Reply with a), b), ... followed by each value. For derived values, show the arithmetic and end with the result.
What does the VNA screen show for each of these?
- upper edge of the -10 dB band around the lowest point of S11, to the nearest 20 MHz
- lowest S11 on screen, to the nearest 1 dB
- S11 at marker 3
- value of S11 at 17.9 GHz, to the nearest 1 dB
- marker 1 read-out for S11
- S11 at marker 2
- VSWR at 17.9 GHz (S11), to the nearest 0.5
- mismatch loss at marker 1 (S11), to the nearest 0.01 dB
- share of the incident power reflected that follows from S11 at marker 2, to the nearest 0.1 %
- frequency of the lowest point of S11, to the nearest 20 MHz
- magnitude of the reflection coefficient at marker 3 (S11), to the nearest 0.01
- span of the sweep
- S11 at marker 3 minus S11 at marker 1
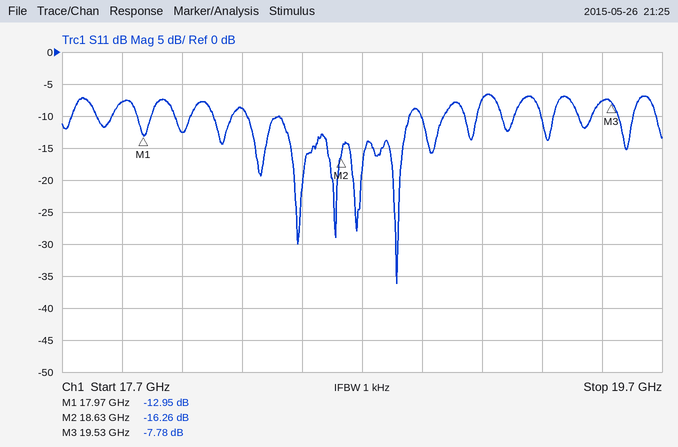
a) 18.86 GHz
b) -36 dB
c) -7.78 dB
d) -8 dB
e) -12.95 dB
f) -16.26 dB
g) |Γ| = 10^(-8/20) = 0.3981; VSWR = (1 + 0.3981)/(1 − 0.3981) ≈ 2.32, so 2.5 to the nearest 0.5
h) −10 log10(1 − 10^(-12.95/10)) ≈ 0.23 dB
i) 10^(-16.26/10) ≈ 2.4 %
j) 18.82 GHz
k) 10^(-7.78/20) ≈ 0.41
l) 2 GHz
m) -7.78 − (-12.95) = 5.17 dB
